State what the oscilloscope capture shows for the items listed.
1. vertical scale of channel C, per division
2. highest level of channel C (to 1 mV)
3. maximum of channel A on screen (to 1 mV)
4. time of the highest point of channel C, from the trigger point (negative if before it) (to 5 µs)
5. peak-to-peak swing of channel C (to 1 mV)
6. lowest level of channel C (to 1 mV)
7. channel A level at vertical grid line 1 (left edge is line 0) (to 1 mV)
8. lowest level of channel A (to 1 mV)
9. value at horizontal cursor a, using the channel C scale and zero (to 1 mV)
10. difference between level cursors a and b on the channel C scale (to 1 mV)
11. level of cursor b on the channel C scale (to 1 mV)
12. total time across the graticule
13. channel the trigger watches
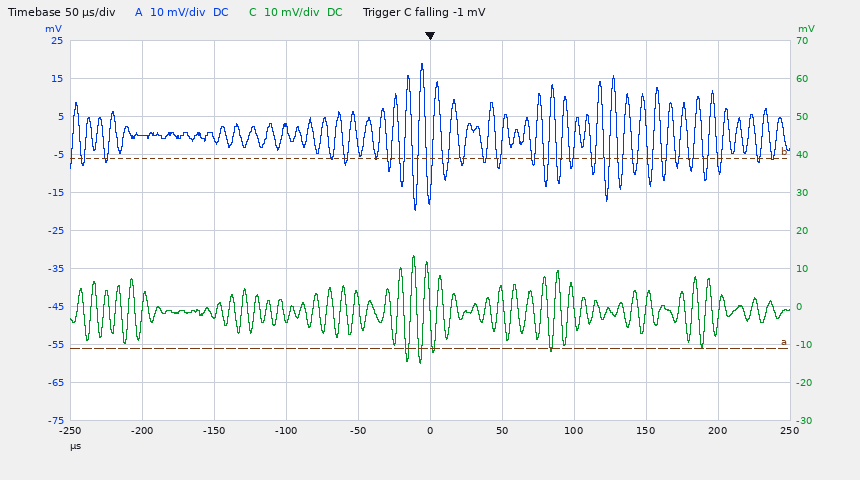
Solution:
10 mV
13 mV
19 mV
-10 µs
28 mV
-15 mV
0 mV
-20 mV
-11 mV
50 mV
39 mV
500 µs
channel C
